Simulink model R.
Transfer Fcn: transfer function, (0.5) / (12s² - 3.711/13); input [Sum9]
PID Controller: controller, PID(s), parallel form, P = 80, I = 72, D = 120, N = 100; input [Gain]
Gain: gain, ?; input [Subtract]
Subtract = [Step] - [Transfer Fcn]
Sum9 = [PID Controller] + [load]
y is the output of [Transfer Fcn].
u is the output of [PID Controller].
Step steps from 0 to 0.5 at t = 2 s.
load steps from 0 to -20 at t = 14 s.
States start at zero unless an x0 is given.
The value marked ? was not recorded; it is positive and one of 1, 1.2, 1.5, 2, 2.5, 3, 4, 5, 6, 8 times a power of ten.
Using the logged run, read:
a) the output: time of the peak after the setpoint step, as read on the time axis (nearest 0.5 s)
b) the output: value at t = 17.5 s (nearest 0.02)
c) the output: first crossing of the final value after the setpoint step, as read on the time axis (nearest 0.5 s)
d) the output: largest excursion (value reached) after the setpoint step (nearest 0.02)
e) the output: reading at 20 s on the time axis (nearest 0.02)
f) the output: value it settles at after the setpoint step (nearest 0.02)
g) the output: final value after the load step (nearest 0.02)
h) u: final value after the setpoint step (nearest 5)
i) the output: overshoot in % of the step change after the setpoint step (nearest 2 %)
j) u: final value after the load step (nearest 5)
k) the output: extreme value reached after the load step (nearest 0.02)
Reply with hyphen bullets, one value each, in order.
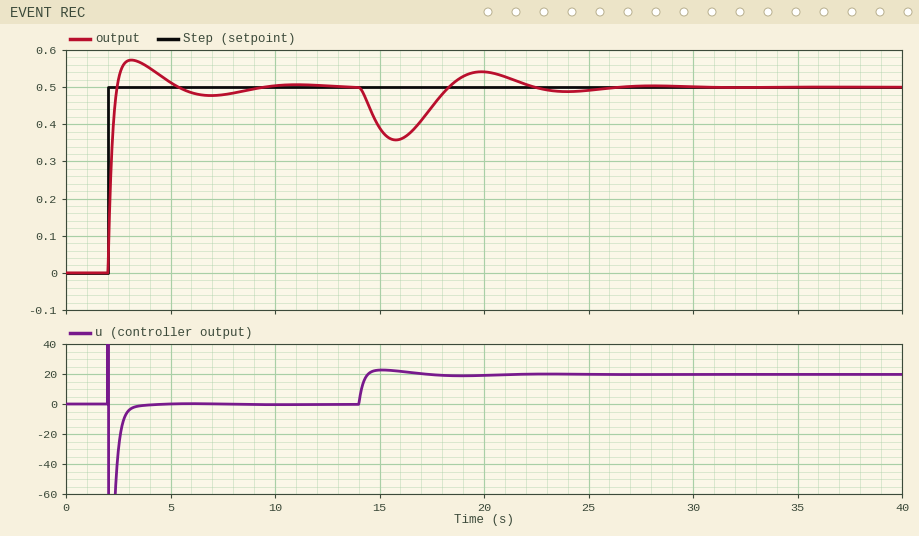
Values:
- 3.0 s
- 0.44
- 2.5 s
- 0.58
- 0.54
- 0.50
- 0.50
- 0
- 14 %
- 20
- 0.36
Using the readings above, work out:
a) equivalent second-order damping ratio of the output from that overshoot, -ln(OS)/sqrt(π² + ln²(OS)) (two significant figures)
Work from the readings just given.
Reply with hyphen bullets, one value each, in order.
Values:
- 0.53
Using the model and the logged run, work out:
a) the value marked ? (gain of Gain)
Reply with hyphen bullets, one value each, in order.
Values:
- 1
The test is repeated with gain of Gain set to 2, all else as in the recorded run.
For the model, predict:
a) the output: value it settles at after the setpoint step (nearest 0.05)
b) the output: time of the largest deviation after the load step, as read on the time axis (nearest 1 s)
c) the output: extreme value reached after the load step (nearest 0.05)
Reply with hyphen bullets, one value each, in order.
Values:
- 0.50
- 16 s
- 0.45
